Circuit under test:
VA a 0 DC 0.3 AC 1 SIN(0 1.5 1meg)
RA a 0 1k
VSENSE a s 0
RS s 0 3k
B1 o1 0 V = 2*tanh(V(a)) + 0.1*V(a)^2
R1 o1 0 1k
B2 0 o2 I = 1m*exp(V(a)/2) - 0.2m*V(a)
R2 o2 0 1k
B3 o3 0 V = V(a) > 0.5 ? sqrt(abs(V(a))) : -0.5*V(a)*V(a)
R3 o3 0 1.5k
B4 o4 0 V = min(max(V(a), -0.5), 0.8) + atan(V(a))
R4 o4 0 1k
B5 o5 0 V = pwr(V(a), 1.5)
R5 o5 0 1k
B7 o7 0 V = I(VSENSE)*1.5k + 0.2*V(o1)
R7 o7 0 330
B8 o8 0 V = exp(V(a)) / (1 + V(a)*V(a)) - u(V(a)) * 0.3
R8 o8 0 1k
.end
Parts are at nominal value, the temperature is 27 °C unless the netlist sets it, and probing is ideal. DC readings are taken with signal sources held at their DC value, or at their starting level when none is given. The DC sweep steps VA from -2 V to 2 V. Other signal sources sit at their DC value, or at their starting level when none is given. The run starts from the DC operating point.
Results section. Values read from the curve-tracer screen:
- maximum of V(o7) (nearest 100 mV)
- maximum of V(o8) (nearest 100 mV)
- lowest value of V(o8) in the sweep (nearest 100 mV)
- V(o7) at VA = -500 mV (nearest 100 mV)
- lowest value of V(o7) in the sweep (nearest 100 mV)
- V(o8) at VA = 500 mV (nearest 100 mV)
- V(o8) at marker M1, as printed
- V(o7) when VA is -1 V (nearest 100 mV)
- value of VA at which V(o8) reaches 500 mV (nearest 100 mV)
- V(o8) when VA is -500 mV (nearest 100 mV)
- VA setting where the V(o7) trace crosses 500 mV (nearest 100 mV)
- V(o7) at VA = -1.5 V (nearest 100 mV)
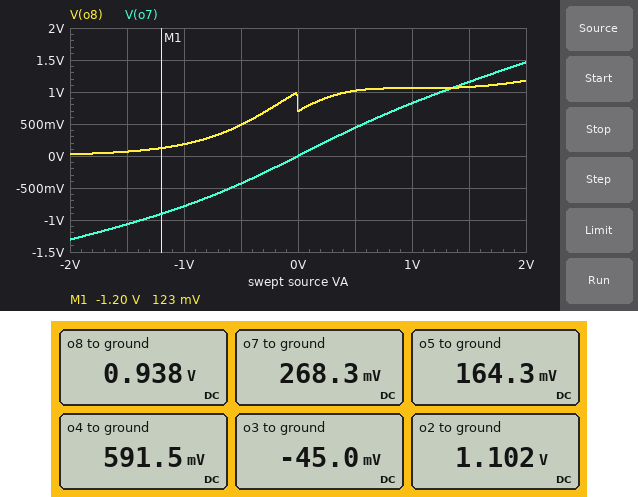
1.5 V
1.2 V
0 V
-400 mV
-1.3 V
1.0 V
123 mV
-800 mV
-500 mV
500 mV
600 mV
-1.1 V
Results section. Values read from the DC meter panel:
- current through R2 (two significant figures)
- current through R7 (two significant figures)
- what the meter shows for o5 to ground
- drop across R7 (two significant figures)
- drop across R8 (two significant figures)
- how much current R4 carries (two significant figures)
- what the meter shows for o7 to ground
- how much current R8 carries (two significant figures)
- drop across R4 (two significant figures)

1.1 mA
810 µA
164.3 mV
270 mV
940 mV
590 µA
268.3 mV
940 µA
590 mV
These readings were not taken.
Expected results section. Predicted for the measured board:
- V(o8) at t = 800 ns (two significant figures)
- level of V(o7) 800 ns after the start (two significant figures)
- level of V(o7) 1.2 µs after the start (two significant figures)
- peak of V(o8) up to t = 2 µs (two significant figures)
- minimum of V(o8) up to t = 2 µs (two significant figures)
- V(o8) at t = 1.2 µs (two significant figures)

79 mV
-1.0 V
1.1 V
1.1 V
69 mV
1.1 V
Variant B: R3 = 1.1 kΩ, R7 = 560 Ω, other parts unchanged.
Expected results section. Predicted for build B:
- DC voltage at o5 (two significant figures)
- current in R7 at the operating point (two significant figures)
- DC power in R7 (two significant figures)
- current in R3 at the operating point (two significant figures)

160 mV
480 µA
130 µW
41 µA
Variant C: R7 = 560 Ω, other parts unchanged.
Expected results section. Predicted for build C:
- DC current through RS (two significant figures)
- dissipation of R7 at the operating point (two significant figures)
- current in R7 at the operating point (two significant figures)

100 µA
130 µW
480 µA
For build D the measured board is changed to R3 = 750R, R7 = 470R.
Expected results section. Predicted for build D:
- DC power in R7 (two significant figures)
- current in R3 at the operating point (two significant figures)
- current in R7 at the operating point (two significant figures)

150 µW
60 µA
570 µA
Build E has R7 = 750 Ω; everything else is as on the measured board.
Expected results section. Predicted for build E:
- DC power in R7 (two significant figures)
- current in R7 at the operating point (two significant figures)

96 µW
360 µA
